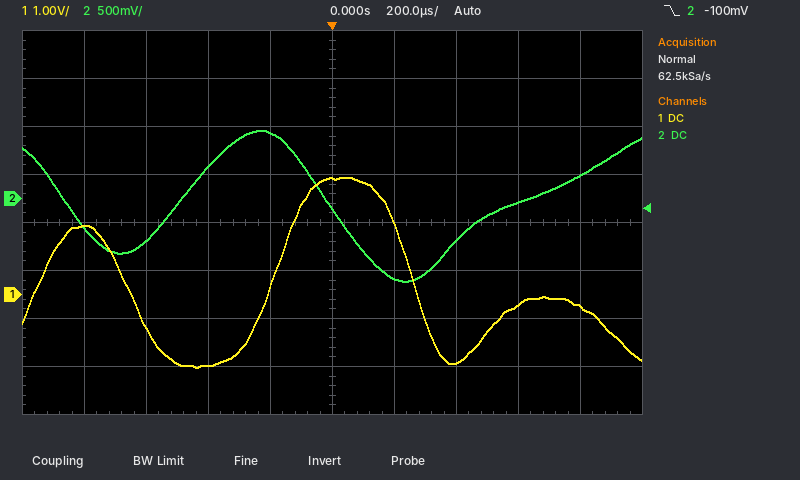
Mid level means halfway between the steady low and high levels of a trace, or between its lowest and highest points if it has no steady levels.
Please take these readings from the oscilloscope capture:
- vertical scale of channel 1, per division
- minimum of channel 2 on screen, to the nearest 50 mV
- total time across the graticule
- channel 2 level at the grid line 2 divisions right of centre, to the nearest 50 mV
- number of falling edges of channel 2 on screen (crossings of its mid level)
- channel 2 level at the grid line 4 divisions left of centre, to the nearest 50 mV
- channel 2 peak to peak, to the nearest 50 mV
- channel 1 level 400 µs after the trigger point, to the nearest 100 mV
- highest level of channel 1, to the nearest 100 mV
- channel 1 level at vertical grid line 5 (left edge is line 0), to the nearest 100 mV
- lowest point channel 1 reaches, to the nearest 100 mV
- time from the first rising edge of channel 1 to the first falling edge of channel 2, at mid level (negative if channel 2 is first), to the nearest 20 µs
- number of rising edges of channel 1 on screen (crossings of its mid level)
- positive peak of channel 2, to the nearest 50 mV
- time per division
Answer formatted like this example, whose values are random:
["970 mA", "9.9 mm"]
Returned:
["1 V", "-850 mV", "2 ms", "-450 mV", "2", "-300 mV", "1.55 V", "-1.4 V", "2.4 V", "2.4 V", "-1.5 V", "+80 µs", "2", "700 mV", "200 µs"]
